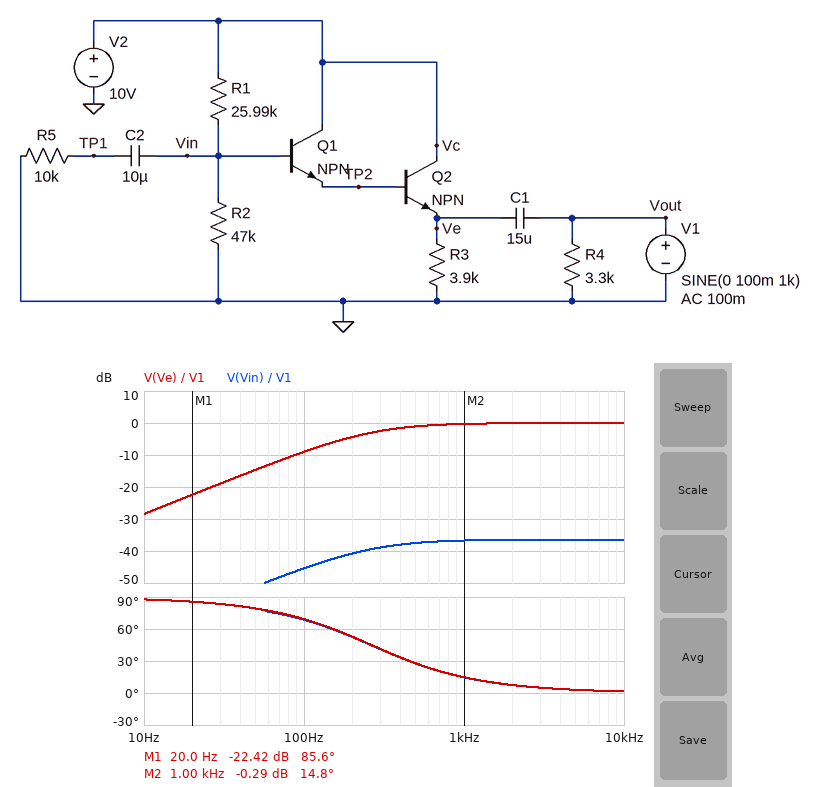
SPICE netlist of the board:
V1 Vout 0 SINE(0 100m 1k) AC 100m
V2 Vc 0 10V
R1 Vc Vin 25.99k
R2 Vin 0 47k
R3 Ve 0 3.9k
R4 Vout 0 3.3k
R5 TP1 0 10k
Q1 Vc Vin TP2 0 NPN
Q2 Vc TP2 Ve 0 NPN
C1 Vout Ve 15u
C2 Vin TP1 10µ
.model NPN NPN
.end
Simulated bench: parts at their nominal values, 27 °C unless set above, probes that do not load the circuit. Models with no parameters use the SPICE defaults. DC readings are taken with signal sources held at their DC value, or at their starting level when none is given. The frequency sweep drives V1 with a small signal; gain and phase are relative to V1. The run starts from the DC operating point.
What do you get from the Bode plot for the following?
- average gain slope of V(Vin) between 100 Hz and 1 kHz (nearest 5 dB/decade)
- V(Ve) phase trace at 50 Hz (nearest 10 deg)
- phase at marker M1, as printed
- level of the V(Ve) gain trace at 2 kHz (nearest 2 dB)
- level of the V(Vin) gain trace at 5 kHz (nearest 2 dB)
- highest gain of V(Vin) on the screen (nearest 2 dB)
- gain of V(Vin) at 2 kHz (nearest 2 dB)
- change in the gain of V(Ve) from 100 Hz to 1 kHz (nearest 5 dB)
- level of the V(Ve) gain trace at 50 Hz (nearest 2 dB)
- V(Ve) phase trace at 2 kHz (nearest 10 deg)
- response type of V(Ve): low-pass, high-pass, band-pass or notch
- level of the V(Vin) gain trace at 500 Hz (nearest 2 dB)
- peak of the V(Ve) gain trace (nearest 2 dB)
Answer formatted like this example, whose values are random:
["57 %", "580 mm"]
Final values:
["10 dB/decade", "80 deg", "85.6 deg", "0 dB", "-36 dB", "-36 dB", "-36 dB", "10 dB", "-14 dB", "10 deg", "high-pass", "-38 dB", "0 dB"]
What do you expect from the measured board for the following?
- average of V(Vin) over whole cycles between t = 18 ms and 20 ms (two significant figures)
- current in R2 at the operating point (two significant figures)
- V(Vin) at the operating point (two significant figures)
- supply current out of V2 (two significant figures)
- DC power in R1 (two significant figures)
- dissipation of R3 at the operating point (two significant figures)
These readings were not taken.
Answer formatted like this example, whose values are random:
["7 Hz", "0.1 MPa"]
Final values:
["6.4 V", "140 µA", "6.4 V", "1.4 mA", "490 µW", "6.4 mW"]
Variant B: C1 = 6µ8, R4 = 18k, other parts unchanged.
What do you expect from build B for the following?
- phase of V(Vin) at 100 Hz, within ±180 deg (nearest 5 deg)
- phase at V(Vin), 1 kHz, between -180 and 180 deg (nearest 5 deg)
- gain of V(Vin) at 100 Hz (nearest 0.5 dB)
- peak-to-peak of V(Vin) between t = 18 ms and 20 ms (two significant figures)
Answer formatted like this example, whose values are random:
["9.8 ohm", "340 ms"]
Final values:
["80 deg", "30 deg", "-52.0 dB", "2.2 mV"]
